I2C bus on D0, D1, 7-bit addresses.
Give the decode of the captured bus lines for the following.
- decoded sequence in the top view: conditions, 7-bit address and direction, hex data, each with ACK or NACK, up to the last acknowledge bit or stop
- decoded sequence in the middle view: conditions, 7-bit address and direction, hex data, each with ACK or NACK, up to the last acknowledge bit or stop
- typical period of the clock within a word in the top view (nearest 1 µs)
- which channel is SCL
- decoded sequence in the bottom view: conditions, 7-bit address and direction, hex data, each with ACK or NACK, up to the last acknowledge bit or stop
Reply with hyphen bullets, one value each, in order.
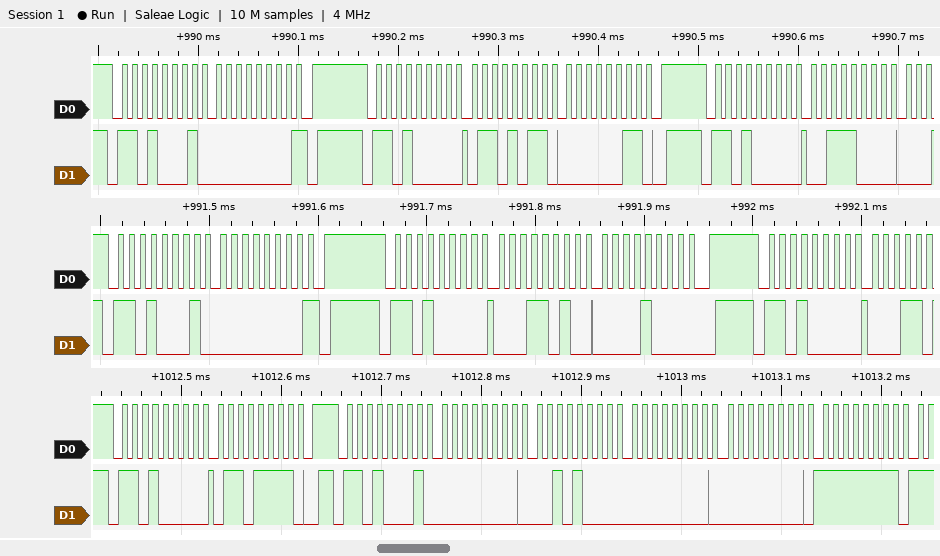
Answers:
- start, address 68 read ACK, 00 NACK, stop, start, address 68 write ACK, 6B ACK, 03 ACK, stop, start, address 68 write ACK, 38 ACK
- start, address 68 read ACK, 00 NACK, stop, start, address 68 write ACK, 1A ACK, 08 ACK, stop, start, address 68 write ACK
- 10 µs
- D0
- start, address 68 write ACK, 6F ACK, stop, start, address 68 read ACK, 00 ACK, 28 ACK, 00 ACK, 00 ACK, FF ACK
